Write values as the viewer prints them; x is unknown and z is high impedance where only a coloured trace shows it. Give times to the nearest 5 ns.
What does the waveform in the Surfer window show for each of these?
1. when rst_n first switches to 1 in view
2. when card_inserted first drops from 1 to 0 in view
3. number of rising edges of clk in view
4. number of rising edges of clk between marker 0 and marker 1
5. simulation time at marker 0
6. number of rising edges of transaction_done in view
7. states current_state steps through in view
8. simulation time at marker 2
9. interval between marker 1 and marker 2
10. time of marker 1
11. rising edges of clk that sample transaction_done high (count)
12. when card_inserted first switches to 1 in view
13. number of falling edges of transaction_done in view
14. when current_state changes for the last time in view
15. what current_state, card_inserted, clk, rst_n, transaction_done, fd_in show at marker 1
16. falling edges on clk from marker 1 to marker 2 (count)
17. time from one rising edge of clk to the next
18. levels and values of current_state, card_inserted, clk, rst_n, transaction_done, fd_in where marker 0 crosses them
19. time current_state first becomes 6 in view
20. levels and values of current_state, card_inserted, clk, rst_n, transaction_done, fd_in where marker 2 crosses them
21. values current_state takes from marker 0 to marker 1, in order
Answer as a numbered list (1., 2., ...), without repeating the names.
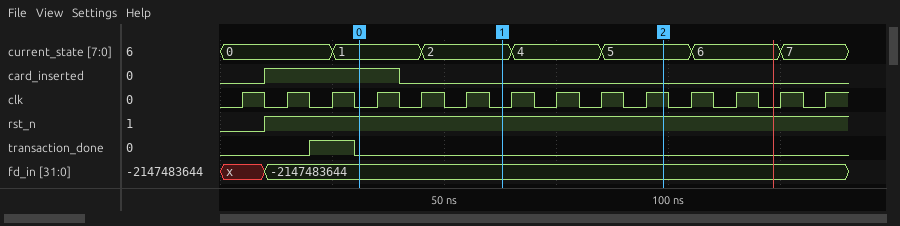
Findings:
1. 10 ns
2. 40 ns
3. 14
4. 3
5. 30 ns
6. 1
7. 0, 1, 2, 4, 5, 6, 7
8. 100 ns
9. 35 ns
10. 65 ns
11. 1
12. 10 ns
13. 1
14. 125 ns
15. current_state=2, card_inserted=0, clk=0, rst_n=1, transaction_done=0, fd_in=-2147483644
16. 3
17. 10 ns
18. current_state=1, card_inserted=1, clk=0, rst_n=1, transaction_done=0, fd_in=-2147483644
19. 105 ns
20. current_state=5, card_inserted=0, clk=1, rst_n=1, transaction_done=0, fd_in=-2147483644
21. 1, 2
